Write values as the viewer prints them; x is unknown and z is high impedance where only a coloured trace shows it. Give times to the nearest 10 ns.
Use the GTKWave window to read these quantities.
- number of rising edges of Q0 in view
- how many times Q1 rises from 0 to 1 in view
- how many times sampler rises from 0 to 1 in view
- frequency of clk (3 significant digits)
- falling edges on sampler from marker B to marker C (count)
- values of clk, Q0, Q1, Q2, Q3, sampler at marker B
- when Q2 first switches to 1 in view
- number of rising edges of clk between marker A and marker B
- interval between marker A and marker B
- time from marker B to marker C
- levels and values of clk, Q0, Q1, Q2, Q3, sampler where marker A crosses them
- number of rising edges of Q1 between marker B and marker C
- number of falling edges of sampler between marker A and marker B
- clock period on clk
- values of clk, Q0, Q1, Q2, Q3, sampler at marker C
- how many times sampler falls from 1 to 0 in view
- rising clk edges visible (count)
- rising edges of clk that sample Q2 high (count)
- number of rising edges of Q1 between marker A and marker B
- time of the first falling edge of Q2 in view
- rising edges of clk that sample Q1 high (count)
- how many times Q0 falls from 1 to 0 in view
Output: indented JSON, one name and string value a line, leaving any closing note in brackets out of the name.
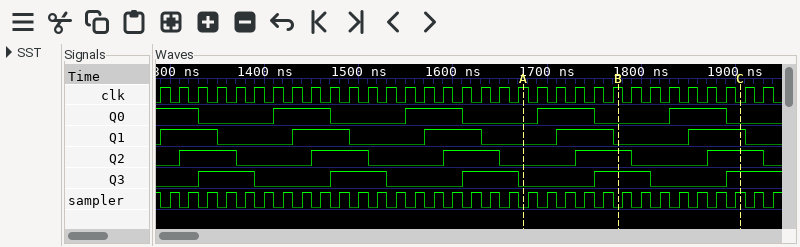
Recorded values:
{
  "number of rising edges of Q0 in view": "4",
  "how many times Q1 rises from 0 to 1 in view": "5",
  "how many times sampler rises from 0 to 1 in view": "33",
  "frequency of clk": "50.0 MHz",
  "falling edges on sampler from marker B to marker C": "6",
  "values of clk, Q0, Q1, Q2, Q3, sampler at marker B": "clk=1, Q0=0, Q1=0, Q2=1, Q3=1, sampler=0",
  "when Q2 first switches to 1 in view": "1310 ns",
  "number of rising edges of clk between marker A and marker B": "5",
  "interval between marker A and marker B": "100 ns",
  "time from marker B to marker C": "130 ns",
  "levels and values of clk, Q0, Q1, Q2, Q3, sampler where marker A crosses them": "clk=1, Q0=0, Q1=0, Q2=0, Q3=0, sampler=0",
  "number of rising edges of Q1 between marker B and marker C": "1",
  "number of falling edges of sampler between marker A and marker B": "5",
  "clock period on clk": "20 ns",
  "values of clk, Q0, Q1, Q2, Q3, sampler at marker C": "clk=0, Q0=0, Q1=1, Q2=1, Q3=1, sampler=1",
  "how many times sampler falls from 1 to 0 in view": "33",
  "rising clk edges visible": "33",
  "rising edges of clk that sample Q2 high": "15",
  "number of rising edges of Q1 between marker A and marker B": "1",
  "time of the first falling edge of Q2 in view": "1370 ns",
  "rising edges of clk that sample Q1 high": "15",
  "how many times Q0 falls from 1 to 0 in view": "5"
}
